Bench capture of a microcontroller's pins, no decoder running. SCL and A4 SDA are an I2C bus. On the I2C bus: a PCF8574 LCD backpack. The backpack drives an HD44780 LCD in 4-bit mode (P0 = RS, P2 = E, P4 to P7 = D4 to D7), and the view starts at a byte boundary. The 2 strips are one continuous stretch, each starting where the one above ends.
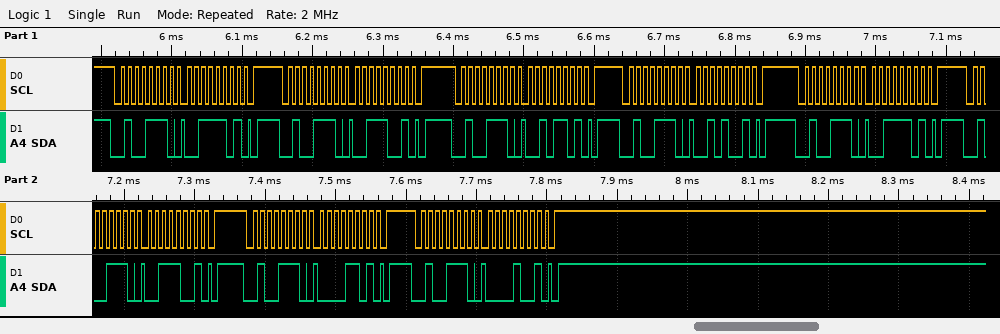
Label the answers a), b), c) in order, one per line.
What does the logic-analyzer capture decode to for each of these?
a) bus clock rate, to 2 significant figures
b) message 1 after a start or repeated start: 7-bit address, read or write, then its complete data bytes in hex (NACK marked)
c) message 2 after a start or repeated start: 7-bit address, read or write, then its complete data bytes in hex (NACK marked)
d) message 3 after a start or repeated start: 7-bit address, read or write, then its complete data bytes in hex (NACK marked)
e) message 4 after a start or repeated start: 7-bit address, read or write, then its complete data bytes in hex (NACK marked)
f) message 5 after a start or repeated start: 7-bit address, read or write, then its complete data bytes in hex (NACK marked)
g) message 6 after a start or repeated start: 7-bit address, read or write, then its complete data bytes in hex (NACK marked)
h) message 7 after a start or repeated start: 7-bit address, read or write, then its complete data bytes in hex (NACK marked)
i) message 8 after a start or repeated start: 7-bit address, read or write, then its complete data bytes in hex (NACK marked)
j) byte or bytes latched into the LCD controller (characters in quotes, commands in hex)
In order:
a) 100 kHz
b) 0x27 write: 3D
c) 0x27 write: 39
d) 0x27 write: 2D
e) 0x27 write: 29
f) 0x27 write: 3D
g) 0x27 write: 39
h) 0x27 write: 0D
i) 0x27 write: 09
j) '2' '0'
